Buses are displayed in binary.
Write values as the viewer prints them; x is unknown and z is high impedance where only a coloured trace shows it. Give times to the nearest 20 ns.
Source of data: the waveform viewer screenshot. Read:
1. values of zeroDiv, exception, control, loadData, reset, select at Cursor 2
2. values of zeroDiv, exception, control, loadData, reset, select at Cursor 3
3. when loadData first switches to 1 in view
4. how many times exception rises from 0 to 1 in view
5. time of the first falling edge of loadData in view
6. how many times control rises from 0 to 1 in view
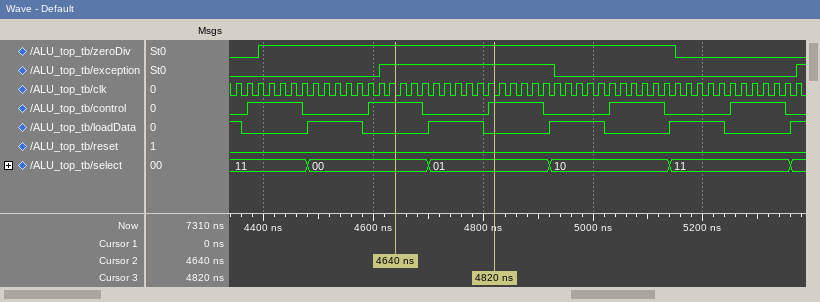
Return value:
zeroDiv=1, exception=1, control=1, loadData=0, reset=0, select=00
zeroDiv=1, exception=1, control=1, loadData=0, reset=0, select=01
4480 ns
2
4360 ns
5
